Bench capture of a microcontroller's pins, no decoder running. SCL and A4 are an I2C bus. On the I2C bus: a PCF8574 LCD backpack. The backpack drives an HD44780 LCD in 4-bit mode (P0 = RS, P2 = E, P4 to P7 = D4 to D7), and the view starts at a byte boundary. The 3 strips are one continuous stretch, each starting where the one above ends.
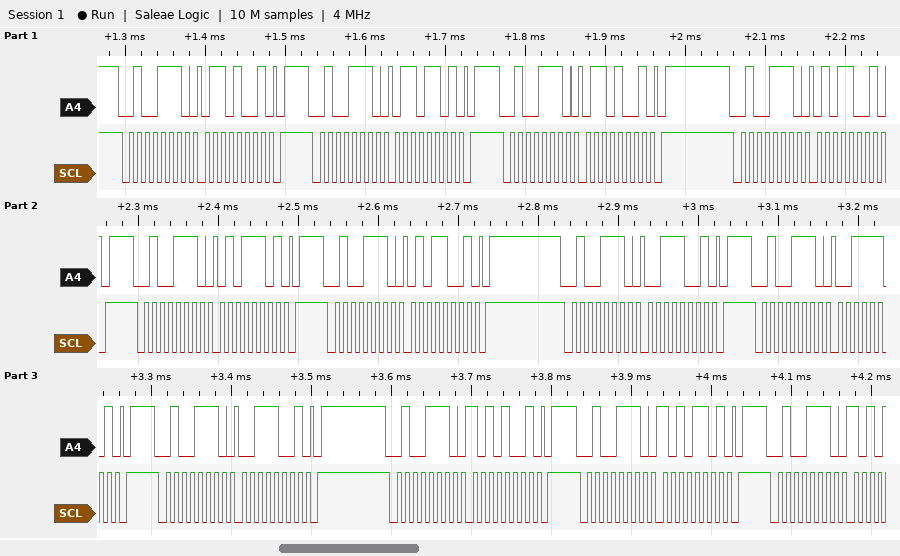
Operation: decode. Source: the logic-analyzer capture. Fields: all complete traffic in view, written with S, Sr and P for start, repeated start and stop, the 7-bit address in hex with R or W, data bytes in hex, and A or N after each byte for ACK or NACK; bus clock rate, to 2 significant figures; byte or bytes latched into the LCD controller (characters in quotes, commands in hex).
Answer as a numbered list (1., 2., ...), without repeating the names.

1. S 27W A 69 A P S 27W A 6D A P S 27W A 69 A P S 27W A 59 A P S 27W A 5D A P S 27W A 59 A P S 27W A 39 A P S 27W A 3D A P S 27W A 39 A P S 27W A A9 A P S 27W A AD A P S 27W A
2. 100 kHz
3. 'e'
